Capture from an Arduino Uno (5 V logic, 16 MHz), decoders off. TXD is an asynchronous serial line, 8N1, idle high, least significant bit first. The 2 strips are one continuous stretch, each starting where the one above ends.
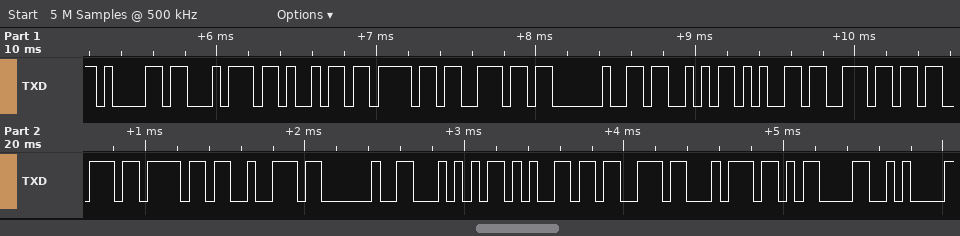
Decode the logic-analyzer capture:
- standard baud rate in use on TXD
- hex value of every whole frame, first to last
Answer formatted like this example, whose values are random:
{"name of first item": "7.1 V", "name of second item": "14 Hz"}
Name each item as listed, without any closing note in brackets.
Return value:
{"standard baud rate in use on TXD": "19200 baud", "hex value of every whole frame, first to last": "0x61 0x74 0x69 0x6F 0x6E 0x20 0x53 0x65 0x6E 0x73 0x6F 0x72 0x20 0x54 0x65 0x73 0x74 0x0D 0x0A"}
